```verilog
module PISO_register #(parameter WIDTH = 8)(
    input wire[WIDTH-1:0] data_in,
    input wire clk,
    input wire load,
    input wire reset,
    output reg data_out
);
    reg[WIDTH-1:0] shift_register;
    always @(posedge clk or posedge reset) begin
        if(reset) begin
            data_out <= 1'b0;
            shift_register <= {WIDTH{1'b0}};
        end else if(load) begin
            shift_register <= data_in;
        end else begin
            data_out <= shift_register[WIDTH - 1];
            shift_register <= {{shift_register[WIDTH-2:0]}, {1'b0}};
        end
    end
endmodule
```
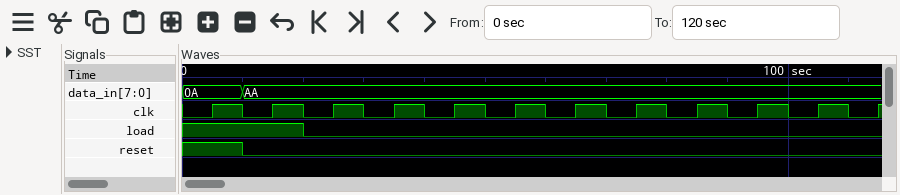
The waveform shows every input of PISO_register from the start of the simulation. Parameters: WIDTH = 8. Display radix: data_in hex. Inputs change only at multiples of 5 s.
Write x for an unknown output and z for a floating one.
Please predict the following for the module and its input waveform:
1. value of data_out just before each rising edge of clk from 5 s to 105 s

0 0 0 1 0 1 0 1 0 1 0
